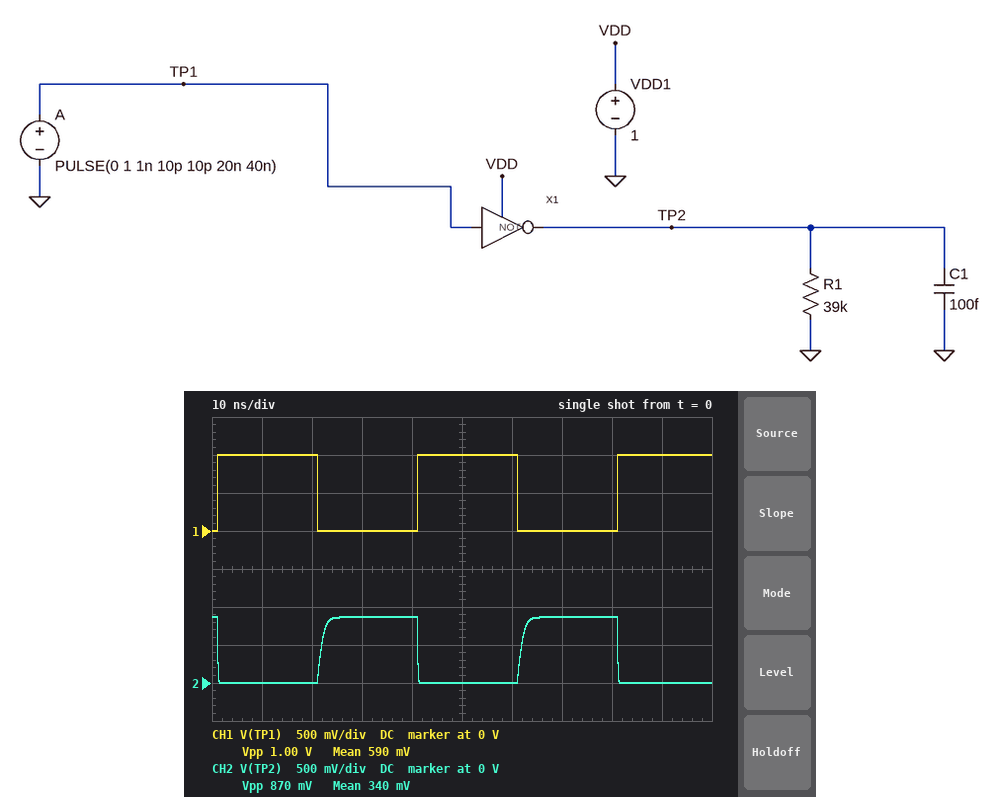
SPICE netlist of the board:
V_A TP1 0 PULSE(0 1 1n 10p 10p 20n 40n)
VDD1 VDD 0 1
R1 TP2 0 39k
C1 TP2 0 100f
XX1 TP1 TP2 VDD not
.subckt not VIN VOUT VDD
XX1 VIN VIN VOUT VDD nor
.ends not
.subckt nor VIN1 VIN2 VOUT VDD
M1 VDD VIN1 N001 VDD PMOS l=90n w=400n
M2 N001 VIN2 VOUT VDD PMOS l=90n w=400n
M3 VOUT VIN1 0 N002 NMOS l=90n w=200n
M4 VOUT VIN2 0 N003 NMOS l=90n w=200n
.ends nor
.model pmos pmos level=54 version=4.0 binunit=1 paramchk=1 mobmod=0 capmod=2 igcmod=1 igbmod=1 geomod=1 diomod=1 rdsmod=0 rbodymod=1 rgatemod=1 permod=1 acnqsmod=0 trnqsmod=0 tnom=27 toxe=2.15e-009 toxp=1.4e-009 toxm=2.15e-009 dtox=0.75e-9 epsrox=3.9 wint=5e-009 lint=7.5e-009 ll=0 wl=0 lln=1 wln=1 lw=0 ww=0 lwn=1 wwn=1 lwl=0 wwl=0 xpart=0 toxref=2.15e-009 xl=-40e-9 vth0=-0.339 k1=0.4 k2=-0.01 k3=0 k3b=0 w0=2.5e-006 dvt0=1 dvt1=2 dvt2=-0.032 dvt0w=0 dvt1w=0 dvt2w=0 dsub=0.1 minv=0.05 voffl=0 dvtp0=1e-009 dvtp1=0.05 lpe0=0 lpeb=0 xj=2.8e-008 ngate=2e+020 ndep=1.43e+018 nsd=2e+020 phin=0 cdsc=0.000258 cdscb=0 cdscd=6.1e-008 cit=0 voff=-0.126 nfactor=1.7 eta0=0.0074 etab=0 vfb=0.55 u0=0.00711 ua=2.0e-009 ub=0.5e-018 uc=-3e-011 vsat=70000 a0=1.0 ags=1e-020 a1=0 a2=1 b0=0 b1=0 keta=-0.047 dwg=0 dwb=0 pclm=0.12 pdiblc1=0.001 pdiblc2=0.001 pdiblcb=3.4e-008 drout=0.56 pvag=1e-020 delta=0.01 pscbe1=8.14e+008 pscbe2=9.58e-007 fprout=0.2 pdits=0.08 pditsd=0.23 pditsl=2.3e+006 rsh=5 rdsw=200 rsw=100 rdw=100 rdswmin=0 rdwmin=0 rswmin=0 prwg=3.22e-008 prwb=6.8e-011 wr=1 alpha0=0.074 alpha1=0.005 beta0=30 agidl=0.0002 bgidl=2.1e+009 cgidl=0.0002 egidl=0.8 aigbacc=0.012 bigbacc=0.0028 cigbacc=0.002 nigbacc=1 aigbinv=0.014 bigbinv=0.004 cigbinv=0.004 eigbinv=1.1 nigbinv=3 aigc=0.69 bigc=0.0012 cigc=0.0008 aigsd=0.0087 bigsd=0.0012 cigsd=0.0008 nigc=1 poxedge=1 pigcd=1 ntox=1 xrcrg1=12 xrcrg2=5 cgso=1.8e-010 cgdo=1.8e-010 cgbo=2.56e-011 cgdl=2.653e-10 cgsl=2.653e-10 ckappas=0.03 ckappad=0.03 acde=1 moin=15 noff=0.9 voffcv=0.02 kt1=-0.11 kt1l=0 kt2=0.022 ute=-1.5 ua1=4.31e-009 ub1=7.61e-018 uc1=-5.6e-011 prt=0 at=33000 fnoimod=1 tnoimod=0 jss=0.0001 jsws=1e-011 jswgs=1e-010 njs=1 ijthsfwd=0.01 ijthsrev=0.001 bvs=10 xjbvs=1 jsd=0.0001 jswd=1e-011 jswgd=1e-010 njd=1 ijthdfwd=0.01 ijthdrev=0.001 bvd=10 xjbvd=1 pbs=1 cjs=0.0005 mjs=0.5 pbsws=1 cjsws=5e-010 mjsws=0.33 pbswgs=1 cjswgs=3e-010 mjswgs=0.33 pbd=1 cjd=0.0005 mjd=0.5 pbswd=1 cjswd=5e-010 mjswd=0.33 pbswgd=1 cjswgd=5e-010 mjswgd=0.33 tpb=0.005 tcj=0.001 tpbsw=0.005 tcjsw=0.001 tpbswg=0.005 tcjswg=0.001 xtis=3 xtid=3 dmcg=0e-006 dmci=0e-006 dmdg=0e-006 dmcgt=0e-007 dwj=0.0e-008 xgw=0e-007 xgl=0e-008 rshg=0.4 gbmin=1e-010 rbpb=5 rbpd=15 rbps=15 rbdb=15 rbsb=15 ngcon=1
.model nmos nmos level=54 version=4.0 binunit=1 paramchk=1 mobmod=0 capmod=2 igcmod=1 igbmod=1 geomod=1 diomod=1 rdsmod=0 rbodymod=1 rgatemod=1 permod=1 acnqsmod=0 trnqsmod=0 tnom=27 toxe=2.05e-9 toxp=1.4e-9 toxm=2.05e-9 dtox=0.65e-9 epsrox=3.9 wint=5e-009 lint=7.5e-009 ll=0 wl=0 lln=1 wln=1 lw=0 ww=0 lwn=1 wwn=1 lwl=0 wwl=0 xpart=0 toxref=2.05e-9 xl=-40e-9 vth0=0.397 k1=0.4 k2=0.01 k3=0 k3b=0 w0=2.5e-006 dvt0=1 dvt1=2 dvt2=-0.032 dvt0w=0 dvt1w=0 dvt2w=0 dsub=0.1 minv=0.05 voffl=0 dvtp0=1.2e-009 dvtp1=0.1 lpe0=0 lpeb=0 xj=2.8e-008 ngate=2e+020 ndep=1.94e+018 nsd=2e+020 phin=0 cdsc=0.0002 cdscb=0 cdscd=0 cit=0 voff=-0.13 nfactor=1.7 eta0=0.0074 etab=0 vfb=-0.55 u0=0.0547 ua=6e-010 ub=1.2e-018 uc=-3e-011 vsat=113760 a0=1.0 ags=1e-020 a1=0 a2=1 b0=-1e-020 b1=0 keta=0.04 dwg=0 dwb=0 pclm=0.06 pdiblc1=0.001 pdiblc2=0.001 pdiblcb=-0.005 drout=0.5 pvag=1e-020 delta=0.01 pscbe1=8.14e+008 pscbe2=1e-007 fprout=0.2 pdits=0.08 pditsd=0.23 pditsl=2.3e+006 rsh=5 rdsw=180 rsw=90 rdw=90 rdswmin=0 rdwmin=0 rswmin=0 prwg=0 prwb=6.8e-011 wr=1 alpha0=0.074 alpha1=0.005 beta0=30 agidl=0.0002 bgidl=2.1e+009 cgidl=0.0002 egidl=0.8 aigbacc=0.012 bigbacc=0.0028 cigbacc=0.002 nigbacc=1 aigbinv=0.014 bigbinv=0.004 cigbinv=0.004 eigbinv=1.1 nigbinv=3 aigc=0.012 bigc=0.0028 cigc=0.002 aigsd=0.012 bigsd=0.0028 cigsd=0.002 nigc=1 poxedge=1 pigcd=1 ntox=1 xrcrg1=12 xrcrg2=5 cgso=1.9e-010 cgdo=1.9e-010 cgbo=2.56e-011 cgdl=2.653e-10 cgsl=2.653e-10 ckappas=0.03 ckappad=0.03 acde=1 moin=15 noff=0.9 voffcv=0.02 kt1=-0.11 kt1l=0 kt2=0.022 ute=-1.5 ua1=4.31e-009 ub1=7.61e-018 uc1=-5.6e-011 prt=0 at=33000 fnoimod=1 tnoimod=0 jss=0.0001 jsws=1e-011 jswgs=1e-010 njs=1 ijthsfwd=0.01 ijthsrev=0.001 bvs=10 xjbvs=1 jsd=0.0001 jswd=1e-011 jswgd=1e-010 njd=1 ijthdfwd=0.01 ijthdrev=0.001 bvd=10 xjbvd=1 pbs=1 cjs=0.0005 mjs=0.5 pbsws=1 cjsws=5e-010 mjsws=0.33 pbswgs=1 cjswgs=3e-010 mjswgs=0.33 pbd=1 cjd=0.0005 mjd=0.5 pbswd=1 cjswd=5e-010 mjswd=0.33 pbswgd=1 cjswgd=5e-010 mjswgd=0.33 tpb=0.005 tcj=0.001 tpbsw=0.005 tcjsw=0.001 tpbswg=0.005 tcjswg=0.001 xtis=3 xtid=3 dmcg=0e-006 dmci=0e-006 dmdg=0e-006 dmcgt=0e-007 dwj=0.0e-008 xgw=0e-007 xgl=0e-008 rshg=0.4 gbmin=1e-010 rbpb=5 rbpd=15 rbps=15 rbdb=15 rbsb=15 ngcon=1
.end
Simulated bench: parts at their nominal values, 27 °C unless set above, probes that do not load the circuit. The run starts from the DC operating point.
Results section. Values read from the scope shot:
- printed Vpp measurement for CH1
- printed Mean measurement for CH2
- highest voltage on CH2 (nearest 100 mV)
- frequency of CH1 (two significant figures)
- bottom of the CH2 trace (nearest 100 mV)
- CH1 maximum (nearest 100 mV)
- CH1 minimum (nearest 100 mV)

1.00 V
340 mV
900 mV
25 MHz
0 V
1.0 V
0 V
